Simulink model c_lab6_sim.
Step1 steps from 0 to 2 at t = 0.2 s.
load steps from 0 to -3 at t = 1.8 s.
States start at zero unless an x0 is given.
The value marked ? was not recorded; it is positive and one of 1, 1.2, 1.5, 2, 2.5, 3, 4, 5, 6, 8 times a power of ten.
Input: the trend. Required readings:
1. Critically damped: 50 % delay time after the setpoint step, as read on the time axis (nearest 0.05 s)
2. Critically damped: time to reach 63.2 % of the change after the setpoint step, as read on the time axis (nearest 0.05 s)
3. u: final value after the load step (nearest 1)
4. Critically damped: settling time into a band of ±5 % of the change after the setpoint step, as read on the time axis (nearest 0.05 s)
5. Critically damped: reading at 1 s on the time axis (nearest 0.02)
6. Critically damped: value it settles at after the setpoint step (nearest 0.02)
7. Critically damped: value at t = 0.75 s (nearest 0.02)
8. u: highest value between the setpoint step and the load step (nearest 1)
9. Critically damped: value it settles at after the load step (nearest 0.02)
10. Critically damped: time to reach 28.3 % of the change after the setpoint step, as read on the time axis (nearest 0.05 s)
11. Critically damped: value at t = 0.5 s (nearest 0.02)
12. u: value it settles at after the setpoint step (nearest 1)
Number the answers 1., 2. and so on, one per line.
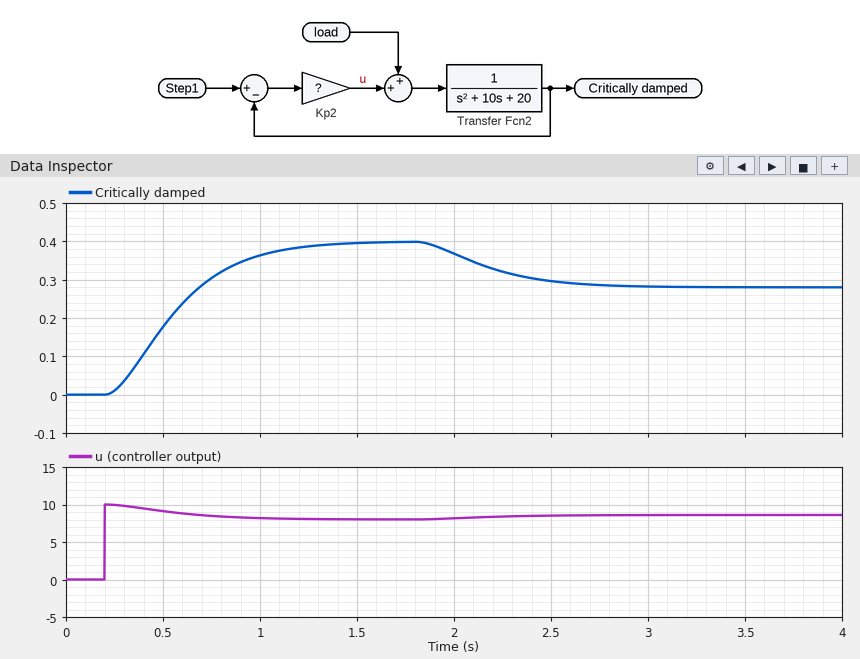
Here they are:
1. 0.55 s
2. 0.65 s
3. 9
4. 1.15 s
5. 0.36
6. 0.40
7. 0.30
8. 10
9. 0.28
10. 0.40 s
11. 0.18
12. 8
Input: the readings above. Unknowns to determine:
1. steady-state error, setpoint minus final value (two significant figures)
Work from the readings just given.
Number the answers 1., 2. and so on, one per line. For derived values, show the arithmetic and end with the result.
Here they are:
1. 2 - 0.4 = 1.6
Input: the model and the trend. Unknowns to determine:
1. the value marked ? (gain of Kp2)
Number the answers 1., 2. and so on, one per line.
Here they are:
1. 5
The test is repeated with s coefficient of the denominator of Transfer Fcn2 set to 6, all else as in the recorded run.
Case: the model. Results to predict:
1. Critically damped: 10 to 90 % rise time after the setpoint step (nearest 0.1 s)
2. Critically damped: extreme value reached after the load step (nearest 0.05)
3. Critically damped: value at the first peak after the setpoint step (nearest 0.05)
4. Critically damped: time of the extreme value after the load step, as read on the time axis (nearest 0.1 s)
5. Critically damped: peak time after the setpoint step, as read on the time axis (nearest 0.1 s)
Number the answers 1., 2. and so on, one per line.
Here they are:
1. 0.4 s
2. 0.25
3. 0.45
4. 2.6 s
5. 1.0 s
